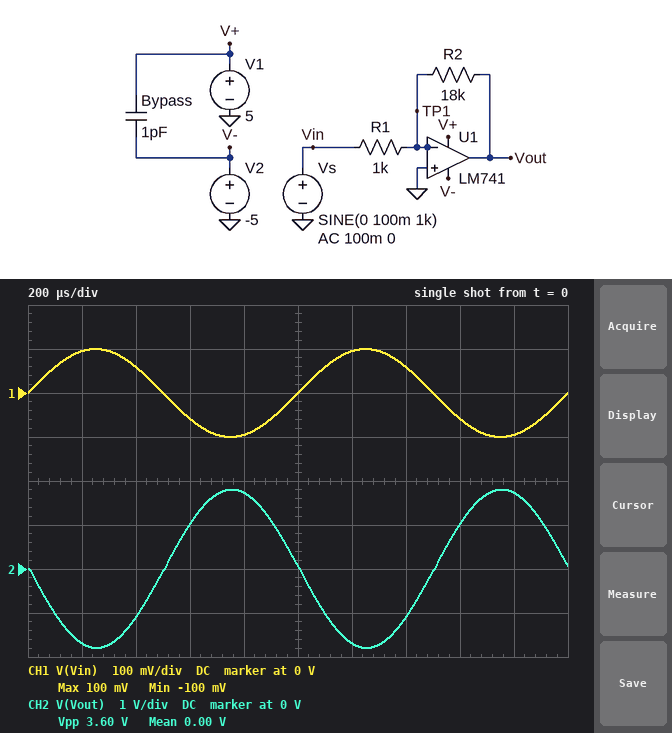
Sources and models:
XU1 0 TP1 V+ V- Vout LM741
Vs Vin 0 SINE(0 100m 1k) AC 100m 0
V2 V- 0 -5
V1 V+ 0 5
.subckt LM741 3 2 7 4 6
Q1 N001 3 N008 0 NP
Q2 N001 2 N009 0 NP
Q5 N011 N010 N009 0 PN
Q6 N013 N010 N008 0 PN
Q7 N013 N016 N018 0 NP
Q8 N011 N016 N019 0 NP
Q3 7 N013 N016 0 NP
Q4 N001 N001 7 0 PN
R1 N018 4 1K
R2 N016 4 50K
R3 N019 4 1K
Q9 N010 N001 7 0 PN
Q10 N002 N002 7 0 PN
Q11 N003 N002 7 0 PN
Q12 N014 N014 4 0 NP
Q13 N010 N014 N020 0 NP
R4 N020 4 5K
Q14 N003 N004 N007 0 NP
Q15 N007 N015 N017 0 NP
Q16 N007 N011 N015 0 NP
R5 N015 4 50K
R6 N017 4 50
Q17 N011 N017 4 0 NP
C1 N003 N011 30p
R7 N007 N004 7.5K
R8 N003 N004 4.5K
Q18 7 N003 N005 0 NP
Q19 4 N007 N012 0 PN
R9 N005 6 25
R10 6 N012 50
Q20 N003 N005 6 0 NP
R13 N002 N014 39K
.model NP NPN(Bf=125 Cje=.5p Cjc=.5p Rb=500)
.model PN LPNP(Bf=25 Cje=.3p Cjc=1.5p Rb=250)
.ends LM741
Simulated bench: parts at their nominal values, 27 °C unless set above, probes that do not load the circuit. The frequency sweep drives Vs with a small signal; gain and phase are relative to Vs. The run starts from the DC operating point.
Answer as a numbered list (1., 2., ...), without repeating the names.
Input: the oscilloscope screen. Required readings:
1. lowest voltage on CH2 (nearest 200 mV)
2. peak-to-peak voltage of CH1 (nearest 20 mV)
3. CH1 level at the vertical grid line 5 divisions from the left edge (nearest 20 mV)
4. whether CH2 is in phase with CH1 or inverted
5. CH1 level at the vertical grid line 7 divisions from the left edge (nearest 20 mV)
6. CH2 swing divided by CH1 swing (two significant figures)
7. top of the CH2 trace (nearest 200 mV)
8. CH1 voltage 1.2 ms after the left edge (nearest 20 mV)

1. -1.8 V
2. 200 mV
3. 0 V
4. inverted
5. 60 mV
6. 18
7. 1.8 V
8. 100 mV
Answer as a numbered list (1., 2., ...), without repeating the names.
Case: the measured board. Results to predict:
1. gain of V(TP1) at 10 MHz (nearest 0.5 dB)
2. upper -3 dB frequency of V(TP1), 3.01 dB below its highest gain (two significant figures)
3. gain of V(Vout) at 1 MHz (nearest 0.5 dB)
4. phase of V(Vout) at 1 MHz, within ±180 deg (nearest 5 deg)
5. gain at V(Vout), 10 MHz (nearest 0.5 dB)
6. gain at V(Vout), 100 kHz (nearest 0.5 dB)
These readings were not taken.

1. -0.5 dB
2. 230 MHz
3. -4.5 dB
4. 25 deg
5. -9.0 dB
6. 9.0 dB
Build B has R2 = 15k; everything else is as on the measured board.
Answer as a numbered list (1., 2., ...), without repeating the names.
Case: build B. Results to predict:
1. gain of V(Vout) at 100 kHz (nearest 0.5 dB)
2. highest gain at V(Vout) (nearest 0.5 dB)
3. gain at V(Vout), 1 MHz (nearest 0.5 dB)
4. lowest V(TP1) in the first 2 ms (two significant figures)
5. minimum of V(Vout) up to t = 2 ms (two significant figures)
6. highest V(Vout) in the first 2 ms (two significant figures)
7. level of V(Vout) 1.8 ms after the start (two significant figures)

1. 8.0 dB
2. 23.5 dB
3. -4.0 dB
4. -4.0 mV
5. -1.5 V
6. 1.5 V
7. 1.4 V
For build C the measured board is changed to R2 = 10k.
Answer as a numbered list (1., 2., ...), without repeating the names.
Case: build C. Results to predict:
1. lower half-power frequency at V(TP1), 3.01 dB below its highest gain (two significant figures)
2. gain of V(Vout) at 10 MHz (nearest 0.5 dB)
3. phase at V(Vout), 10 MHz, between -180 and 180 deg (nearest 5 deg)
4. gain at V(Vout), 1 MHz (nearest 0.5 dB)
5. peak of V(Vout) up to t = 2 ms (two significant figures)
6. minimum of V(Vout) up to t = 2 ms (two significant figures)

1. 19 kHz
2. -5.5 dB
3. -35 deg
4. -3.0 dB
5. 1.0 V
6. -1.0 V
